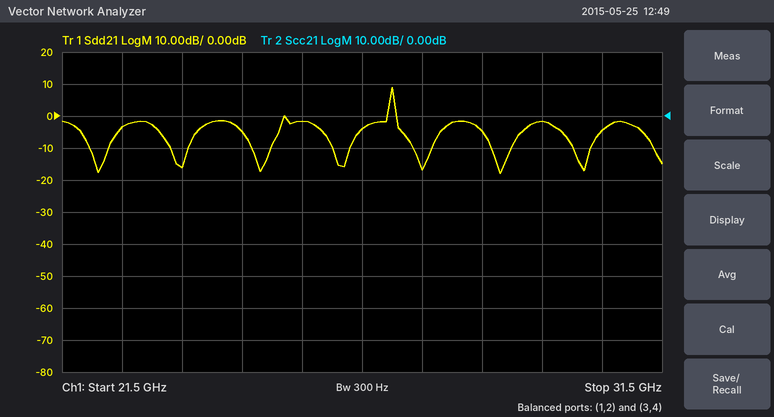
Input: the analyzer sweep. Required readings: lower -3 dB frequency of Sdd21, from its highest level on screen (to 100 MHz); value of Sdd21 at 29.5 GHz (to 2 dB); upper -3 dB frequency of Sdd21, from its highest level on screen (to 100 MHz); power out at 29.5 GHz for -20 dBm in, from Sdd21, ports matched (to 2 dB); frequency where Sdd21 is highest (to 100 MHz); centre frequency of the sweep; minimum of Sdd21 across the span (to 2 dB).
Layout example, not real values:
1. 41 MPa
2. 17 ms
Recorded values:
1. 27.0 GHz
2. -2 dB
3. 27.0 GHz
4. -22 dBm
5. 27.0 GHz
6. 26.5 GHz
7. -18 dB
